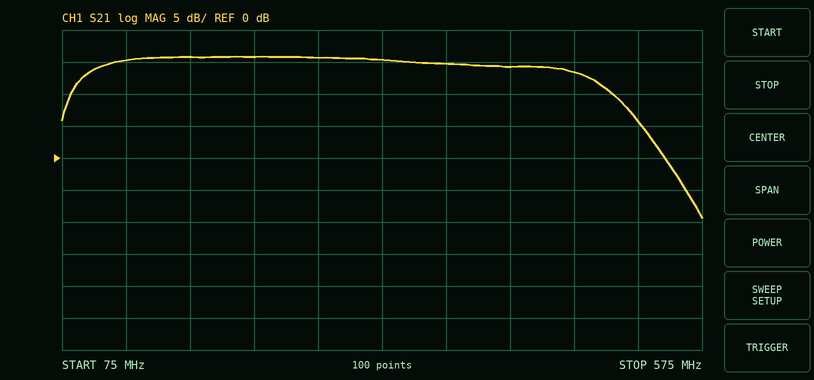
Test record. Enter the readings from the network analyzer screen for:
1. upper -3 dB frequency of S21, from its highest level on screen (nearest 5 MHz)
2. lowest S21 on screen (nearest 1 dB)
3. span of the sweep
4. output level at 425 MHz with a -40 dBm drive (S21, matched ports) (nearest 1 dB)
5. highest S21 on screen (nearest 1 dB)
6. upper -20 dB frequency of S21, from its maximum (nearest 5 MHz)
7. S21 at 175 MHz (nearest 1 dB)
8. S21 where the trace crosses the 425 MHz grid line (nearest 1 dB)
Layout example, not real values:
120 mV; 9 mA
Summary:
485 MHz; -9 dB; 500 MHz; -26 dBm; 16 dB; 560 MHz; 16 dB; 14 dB
